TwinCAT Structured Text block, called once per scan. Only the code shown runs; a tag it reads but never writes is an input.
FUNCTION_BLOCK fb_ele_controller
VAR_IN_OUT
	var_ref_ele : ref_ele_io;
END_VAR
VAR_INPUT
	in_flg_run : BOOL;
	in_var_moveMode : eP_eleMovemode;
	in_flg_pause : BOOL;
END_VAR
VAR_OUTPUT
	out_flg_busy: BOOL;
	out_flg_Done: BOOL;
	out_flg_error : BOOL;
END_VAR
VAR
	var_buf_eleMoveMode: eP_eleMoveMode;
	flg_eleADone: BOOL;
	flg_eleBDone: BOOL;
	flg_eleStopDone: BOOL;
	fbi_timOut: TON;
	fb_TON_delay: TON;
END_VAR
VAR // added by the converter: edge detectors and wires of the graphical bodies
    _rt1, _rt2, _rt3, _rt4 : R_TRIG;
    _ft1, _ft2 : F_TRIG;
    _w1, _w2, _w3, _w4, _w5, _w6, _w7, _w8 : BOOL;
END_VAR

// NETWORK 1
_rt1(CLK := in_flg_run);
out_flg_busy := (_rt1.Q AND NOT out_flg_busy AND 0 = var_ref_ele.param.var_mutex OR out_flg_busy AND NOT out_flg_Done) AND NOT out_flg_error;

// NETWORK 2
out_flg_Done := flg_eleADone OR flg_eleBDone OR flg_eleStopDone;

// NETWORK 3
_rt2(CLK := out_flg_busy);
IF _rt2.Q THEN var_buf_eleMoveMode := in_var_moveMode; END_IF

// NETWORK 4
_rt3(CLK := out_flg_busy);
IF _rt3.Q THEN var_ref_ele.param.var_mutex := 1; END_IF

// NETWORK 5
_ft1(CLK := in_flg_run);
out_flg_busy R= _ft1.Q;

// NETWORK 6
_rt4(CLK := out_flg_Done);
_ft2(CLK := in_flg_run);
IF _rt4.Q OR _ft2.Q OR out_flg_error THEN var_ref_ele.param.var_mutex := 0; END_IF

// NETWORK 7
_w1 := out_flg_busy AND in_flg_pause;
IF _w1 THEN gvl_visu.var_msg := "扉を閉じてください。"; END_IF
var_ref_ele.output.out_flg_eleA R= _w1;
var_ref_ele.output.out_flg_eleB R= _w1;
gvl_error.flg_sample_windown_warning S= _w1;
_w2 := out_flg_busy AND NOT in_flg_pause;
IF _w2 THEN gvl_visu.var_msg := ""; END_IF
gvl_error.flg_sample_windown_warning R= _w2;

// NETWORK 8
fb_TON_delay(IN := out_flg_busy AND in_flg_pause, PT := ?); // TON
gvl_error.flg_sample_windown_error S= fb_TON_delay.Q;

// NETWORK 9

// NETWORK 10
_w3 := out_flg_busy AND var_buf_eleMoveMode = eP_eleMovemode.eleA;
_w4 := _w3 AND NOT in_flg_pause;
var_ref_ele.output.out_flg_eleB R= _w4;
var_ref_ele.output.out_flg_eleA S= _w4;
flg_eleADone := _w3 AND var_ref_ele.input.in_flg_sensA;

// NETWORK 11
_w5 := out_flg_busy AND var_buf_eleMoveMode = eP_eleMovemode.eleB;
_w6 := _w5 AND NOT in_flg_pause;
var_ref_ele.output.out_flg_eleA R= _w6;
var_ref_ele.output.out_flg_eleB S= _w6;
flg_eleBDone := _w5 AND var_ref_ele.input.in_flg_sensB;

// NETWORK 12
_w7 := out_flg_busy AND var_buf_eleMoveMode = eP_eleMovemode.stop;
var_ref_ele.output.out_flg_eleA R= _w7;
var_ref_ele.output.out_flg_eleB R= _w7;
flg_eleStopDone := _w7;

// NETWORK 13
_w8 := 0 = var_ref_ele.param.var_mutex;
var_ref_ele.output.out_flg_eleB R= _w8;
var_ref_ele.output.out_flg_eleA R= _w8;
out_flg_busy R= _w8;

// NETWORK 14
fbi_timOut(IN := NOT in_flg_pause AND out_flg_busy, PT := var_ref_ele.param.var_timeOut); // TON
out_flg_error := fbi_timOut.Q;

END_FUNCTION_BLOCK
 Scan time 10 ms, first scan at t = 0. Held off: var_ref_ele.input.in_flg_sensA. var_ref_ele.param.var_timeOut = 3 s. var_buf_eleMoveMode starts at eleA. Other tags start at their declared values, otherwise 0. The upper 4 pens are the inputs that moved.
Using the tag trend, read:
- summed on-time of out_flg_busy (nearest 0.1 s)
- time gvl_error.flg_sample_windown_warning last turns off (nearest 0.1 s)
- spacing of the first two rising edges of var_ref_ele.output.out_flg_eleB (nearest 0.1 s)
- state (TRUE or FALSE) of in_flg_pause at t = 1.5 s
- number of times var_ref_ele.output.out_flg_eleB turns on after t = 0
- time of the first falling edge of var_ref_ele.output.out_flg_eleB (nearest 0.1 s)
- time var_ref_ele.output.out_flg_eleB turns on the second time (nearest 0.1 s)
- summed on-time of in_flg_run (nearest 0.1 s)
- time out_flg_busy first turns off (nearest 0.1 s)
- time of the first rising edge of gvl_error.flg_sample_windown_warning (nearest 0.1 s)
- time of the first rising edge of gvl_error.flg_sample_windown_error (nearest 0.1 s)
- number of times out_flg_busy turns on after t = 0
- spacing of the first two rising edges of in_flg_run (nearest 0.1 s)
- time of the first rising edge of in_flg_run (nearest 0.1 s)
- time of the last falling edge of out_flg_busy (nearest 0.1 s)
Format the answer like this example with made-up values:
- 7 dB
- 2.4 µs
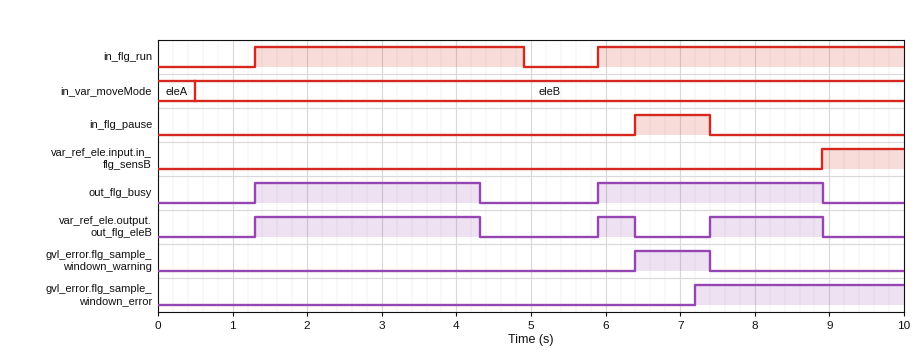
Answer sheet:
- 6.0 s
- 7.4 s
- 4.6 s
- FALSE
- 3
- 4.3 s
- 5.9 s
- 7.7 s
- 4.3 s
- 6.4 s
- 7.2 s
- 2
- 4.6 s
- 1.3 s
- 8.9 s
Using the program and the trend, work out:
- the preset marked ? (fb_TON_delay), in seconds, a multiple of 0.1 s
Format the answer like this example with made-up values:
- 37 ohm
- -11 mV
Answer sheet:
- 0.8 s
